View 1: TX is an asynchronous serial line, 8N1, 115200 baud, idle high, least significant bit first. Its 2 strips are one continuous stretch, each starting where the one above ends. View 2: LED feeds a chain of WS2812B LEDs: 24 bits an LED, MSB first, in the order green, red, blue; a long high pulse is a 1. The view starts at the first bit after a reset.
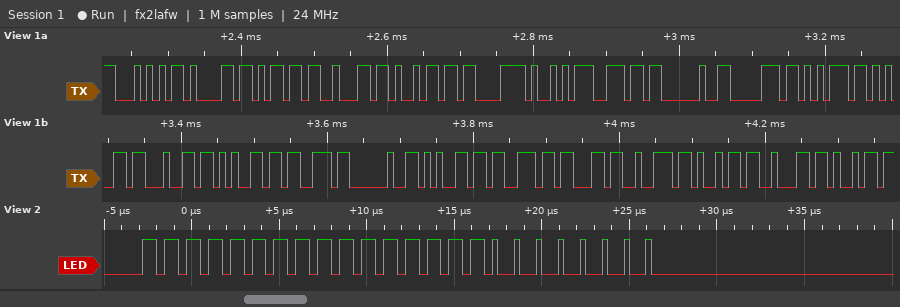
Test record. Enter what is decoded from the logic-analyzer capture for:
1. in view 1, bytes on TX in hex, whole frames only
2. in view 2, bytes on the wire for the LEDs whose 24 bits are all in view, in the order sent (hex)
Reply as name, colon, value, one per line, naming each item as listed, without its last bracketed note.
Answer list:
in view 1, bytes on TX in hex, whole frames only: 54 61 6D 62 69 C3 A9 6E 20 70 75 65 64 65 73 20 65 73 63 72 69 62 69
in view 2, bytes on the wire for the LEDs whose 24 bits are all in view, in the order sent: FF FF 00
